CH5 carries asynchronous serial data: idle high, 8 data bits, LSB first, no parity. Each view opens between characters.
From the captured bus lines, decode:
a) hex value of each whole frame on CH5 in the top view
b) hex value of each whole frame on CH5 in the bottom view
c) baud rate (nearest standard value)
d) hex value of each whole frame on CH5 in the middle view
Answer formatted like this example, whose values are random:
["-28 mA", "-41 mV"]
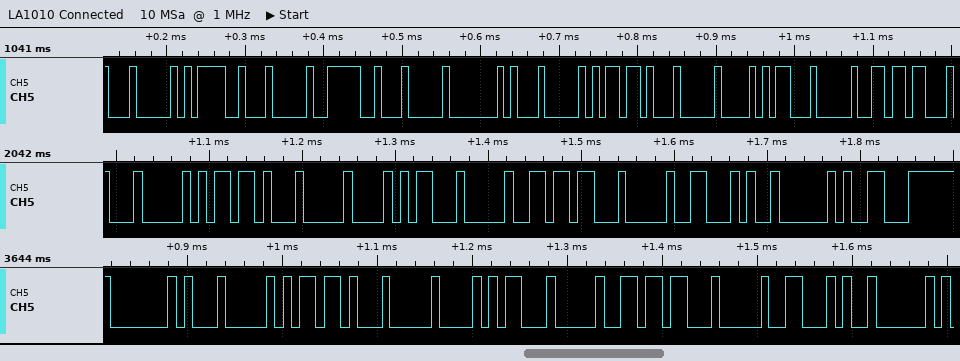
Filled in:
["04, 3D, 04, 3E, 04, 40, 04, 6D, 04, A8, 04, B6", "40, 04, 6D, 04, A8, 04, B6, 04, 46, 02", "115200 baud", "04, 6D, 04, A8, 04, B6, 04, 46, 02, 19"]
